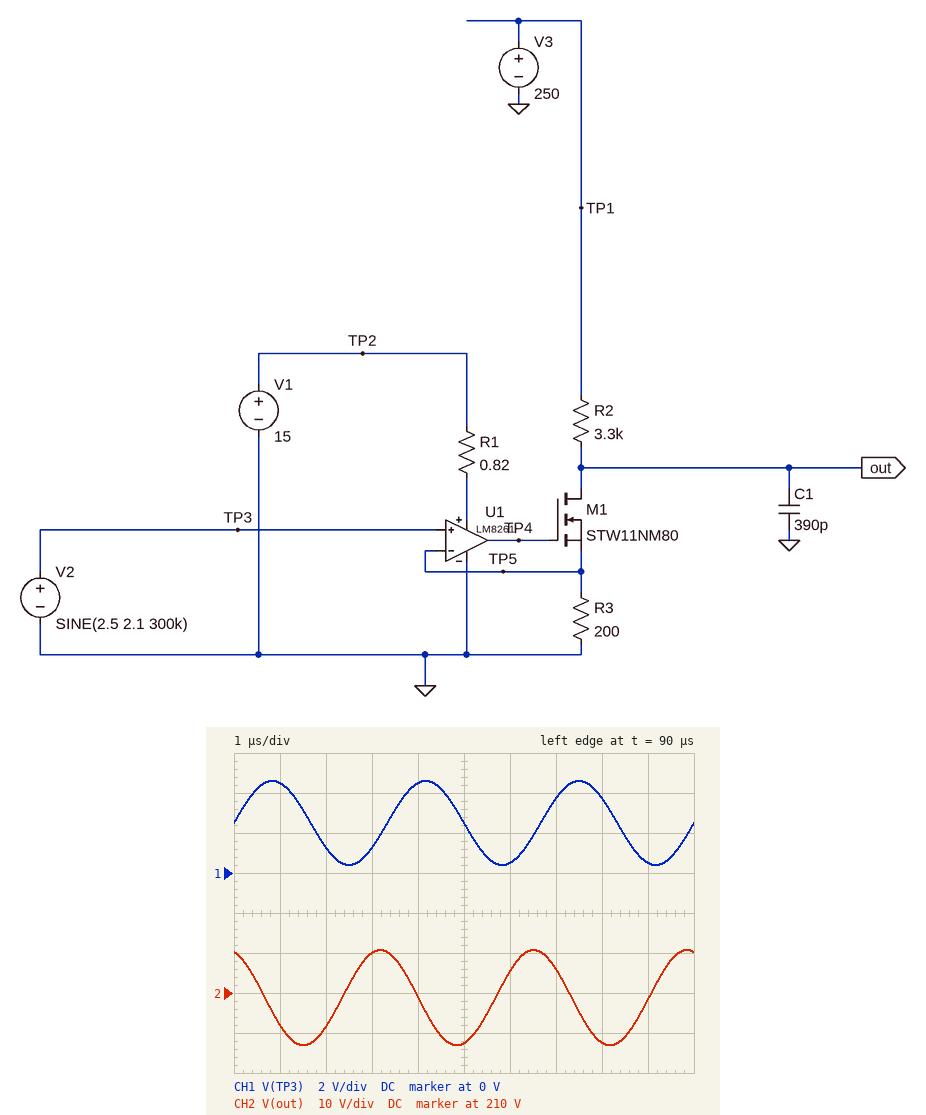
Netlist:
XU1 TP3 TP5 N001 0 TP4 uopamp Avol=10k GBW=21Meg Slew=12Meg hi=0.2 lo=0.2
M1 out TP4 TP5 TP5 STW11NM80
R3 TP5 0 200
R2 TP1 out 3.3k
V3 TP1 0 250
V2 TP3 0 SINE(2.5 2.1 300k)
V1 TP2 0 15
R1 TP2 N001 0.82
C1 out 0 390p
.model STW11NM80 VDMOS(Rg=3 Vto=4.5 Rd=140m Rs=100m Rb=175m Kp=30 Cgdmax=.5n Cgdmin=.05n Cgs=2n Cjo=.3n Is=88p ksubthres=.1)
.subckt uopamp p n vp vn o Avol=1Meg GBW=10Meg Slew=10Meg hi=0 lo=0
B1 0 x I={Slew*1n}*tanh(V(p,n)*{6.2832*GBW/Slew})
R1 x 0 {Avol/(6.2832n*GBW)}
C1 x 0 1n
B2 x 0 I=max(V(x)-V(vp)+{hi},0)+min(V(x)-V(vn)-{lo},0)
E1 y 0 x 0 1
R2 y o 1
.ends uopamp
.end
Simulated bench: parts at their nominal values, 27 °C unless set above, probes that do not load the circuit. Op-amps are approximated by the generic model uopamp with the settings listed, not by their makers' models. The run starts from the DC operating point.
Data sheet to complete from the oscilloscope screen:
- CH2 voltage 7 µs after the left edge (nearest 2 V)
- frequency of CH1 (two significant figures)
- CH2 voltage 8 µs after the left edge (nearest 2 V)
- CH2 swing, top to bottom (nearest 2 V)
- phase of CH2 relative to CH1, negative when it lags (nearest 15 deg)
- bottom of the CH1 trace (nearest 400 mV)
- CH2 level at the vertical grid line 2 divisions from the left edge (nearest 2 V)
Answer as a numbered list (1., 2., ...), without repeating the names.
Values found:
1. 216 V
2. 300 kHz
3. 198 V
4. 24 V
5. 105 deg
6. 400 mV
7. 202 V
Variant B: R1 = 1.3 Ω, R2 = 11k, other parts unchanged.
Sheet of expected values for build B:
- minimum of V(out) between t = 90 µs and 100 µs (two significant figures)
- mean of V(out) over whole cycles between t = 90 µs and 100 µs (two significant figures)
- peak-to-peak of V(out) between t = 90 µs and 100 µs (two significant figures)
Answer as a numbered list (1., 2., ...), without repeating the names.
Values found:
1. 100 V
2. 110 V
3. 25 V
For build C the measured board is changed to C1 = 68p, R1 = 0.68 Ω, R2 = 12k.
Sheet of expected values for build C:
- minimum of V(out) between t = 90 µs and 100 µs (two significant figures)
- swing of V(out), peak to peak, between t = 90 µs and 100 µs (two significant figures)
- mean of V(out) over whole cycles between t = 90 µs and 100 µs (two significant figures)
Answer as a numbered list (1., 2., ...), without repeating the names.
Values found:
1. 57 V
2. 88 V
3. 100 V
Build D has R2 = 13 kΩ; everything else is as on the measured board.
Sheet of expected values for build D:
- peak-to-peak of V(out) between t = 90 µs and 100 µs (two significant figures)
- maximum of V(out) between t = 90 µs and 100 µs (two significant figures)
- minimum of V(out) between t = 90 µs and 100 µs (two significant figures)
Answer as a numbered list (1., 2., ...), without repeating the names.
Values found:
1. 25 V
2. 100 V
3. 75 V
